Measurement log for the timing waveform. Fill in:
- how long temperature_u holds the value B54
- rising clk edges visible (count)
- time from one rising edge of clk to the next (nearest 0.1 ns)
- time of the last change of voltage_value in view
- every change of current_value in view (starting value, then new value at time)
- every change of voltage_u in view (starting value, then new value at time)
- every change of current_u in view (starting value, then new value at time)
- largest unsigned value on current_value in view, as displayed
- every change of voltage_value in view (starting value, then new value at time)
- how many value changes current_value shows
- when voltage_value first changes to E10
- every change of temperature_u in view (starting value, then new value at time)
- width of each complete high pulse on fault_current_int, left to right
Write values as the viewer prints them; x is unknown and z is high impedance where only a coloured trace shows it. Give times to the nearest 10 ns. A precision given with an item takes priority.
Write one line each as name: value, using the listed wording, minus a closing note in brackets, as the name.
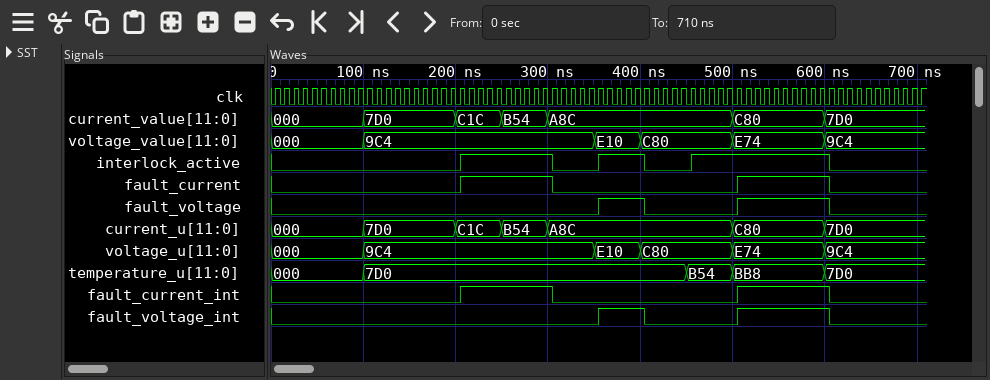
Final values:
how long temperature_u holds the value B54: 50 ns
rising clk edges visible: 71
time from one rising edge of clk to the next: 10 ns
time of the last change of voltage_value in view: 600 ns
every change of current_value in view: 000, 7D0 at 100 ns, C1C at 200 ns, B54 at 250 ns, A8C at 300 ns, C80 at 500 ns, 7D0 at 600 ns
every change of voltage_u in view: 000, 9C4 at 100 ns, E10 at 350 ns, C80 at 400 ns, E74 at 500 ns, 9C4 at 600 ns
every change of current_u in view: 000, 7D0 at 100 ns, C1C at 200 ns, B54 at 250 ns, A8C at 300 ns, C80 at 500 ns, 7D0 at 600 ns
largest unsigned value on current_value in view, as displayed: C80
every change of voltage_value in view: 000, 9C4 at 100 ns, E10 at 350 ns, C80 at 400 ns, E74 at 500 ns, 9C4 at 600 ns
how many value changes current_value shows: 6
when voltage_value first changes to E10: 350 ns
every change of temperature_u in view: 000, 7D0 at 100 ns, B54 at 450 ns, BB8 at 500 ns, 7D0 at 600 ns
width of each complete high pulse on fault_current_int, left to right: 100 ns, 100 ns
